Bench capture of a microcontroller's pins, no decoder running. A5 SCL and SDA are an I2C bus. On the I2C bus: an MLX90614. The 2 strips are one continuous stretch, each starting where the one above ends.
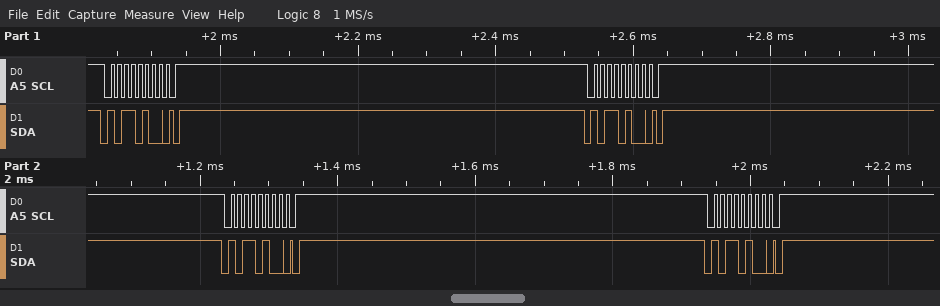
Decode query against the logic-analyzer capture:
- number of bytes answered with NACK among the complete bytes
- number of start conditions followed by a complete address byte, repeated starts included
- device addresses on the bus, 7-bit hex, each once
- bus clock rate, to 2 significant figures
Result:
0
4
0x5A
100 kHz
